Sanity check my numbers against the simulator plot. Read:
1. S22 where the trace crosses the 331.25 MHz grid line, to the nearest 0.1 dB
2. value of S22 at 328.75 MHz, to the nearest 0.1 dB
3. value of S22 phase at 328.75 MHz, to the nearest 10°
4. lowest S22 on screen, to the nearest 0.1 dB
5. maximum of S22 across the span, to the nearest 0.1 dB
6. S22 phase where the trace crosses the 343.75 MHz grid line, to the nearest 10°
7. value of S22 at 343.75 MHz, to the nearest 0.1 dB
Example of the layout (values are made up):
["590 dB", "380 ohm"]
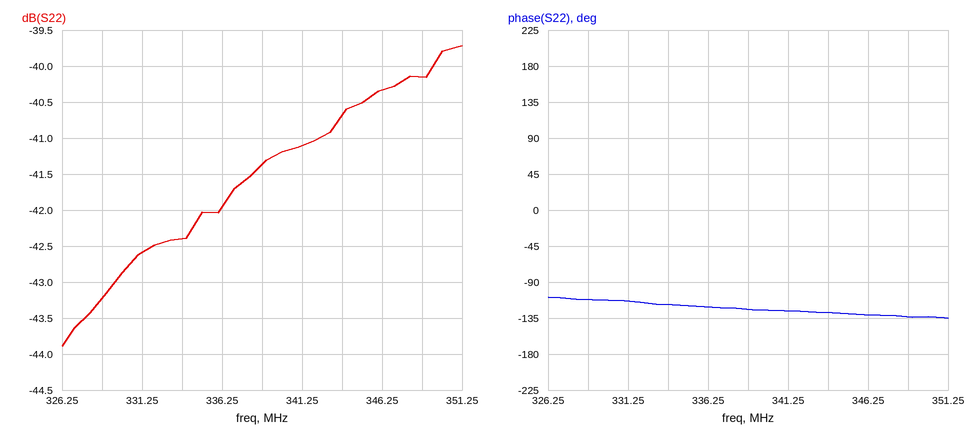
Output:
["-42.6 dB", "-43.2 dB", "-110°", "-43.9 dB", "-39.7 dB", "-130°", "-40.7 dB"]
